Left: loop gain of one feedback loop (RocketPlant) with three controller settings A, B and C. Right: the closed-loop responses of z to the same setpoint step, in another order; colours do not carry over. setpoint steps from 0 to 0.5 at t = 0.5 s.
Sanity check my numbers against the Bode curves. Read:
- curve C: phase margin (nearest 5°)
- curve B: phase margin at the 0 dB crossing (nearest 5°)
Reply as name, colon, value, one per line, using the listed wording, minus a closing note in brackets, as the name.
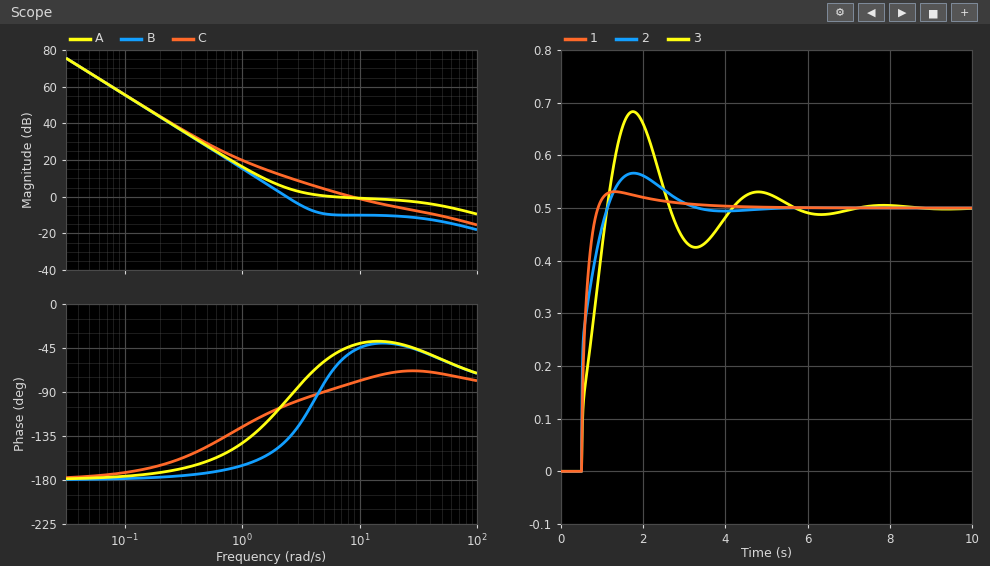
curve C: phase margin: 100°
curve B: phase margin at the 0 dB crossing: 40°
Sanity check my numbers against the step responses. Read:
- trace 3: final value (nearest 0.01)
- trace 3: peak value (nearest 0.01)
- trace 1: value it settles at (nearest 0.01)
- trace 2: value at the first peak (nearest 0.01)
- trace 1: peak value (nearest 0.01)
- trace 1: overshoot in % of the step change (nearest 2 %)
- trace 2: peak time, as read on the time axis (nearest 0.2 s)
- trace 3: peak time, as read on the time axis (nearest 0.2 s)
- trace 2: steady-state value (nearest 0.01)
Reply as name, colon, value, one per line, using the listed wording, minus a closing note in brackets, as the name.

trace 3: final value: 0.50
trace 3: peak value: 0.68
trace 1: value it settles at: 0.50
trace 2: value at the first peak: 0.57
trace 1: peak value: 0.53
trace 1: overshoot in % of the step change: 6 %
trace 2: peak time, as read on the time axis: 1.8 s
trace 3: peak time, as read on the time axis: 1.8 s
trace 2: steady-state value: 0.50
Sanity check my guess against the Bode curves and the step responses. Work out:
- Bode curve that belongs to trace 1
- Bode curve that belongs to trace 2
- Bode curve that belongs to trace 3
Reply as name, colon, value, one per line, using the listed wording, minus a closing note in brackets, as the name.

Bode curve that belongs to trace 1: C
Bode curve that belongs to trace 2: A
Bode curve that belongs to trace 3: B
